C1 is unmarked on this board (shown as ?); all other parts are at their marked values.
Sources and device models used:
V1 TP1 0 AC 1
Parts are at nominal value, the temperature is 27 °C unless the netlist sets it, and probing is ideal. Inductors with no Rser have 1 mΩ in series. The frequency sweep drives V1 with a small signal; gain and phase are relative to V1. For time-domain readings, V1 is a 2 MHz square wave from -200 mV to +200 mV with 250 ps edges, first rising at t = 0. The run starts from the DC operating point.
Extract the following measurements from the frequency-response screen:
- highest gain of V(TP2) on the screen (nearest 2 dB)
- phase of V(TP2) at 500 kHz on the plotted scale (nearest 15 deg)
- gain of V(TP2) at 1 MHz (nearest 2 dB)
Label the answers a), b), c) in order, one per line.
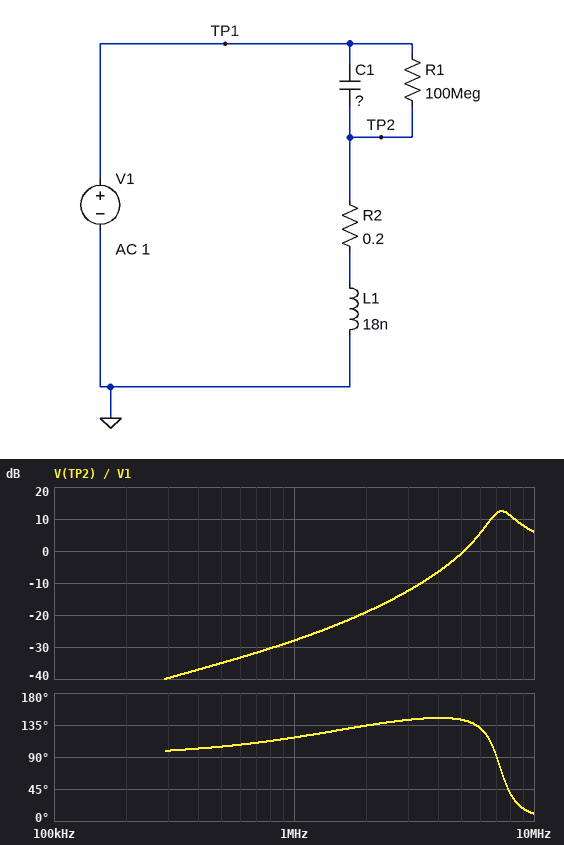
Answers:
a) 12 dB
b) 105 deg
c) -28 dB
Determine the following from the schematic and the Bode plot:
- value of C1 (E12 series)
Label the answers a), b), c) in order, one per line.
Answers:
a) 27 nF
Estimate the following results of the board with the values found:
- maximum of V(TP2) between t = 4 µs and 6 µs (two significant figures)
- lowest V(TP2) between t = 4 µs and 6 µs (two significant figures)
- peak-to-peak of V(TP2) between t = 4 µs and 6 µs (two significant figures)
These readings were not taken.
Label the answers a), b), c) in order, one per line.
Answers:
a) 370 mV
b) -370 mV
c) 740 mV
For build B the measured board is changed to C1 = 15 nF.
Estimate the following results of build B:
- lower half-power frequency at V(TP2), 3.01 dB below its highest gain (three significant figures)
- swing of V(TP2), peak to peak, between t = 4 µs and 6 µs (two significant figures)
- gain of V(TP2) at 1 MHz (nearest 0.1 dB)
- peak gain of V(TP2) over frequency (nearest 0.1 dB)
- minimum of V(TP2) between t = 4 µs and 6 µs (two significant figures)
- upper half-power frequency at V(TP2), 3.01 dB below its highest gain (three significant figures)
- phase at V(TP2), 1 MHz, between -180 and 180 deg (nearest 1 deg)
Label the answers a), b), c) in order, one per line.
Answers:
a) 8.97 MHz
b) 980 mV
c) -33.2 dB
d) 14.9 dB
e) -490 mV
f) 10.8 MHz
g) 118 deg
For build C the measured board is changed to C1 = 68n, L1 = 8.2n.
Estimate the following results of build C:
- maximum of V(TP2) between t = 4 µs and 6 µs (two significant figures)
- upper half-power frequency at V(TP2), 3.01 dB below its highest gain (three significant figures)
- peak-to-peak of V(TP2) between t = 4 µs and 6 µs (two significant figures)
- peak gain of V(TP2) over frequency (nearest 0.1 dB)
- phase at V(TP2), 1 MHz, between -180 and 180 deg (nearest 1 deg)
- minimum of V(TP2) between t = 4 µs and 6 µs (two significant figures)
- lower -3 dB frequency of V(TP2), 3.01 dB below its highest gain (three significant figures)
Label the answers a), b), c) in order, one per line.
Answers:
a) 420 mV
b) 11.3 MHz
c) 840 mV
d) 6.2 dB
e) 99 deg
f) -420 mV
g) 5.56 MHz
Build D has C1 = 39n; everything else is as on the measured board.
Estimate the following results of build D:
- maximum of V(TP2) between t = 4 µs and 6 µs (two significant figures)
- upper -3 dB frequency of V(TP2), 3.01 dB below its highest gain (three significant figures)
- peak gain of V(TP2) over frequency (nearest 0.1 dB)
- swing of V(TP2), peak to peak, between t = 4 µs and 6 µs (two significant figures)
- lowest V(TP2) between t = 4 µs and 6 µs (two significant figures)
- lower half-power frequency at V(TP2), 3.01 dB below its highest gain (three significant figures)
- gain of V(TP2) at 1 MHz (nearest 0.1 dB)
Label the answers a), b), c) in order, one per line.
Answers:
a) 530 mV
b) 7.34 MHz
c) 11.0 dB
d) 1.1 V
e) -530 mV
f) 5.36 MHz
g) -24.7 dB
